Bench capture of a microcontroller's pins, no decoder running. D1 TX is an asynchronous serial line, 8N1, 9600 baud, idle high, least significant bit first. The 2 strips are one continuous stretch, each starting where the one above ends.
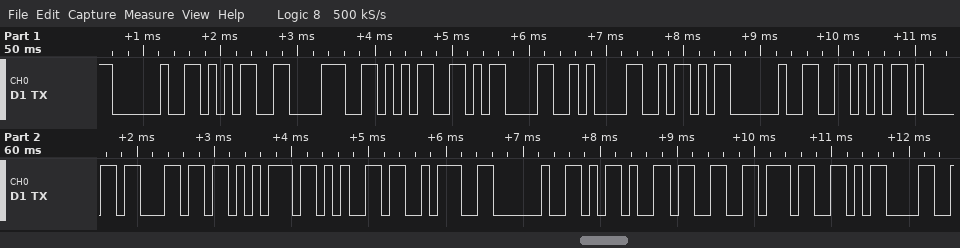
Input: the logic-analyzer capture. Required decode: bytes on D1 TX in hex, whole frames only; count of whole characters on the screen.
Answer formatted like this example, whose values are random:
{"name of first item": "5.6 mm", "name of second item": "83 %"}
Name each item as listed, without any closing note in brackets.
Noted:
{"bytes on D1 TX in hex, whole frames only": "20 35 38 35 0D 0A 5A 20 56 61 6C 75 65 3A 20 2D 33 37 0D", "count of whole characters on the screen": "19"}
